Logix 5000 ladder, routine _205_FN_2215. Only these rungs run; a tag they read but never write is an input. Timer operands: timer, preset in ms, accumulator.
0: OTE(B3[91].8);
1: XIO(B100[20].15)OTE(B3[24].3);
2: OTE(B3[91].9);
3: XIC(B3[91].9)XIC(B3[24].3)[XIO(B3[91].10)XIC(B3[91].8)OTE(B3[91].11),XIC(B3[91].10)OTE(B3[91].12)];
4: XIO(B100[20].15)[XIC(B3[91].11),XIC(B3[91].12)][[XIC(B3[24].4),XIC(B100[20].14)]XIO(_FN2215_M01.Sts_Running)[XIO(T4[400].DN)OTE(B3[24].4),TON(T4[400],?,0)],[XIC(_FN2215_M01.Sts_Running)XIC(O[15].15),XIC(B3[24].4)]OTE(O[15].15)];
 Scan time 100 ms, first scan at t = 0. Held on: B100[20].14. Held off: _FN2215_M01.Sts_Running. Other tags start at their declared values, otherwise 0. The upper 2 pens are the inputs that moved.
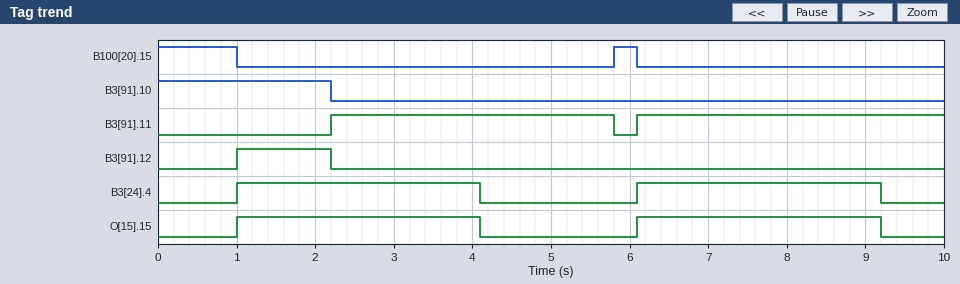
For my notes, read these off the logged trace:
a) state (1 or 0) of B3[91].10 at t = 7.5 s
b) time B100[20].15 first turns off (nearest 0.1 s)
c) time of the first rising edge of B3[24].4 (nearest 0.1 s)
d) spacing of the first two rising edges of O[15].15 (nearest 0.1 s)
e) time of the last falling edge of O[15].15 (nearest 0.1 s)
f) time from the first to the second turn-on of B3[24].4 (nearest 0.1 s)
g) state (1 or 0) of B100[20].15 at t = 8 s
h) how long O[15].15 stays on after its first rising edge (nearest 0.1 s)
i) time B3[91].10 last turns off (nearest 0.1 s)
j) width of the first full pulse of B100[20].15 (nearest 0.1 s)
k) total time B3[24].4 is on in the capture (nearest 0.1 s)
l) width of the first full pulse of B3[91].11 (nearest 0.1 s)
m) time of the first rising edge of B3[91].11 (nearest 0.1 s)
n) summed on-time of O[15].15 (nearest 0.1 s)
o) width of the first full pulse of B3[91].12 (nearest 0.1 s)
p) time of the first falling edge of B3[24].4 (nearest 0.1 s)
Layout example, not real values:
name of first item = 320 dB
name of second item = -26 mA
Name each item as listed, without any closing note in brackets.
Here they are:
state (1 or 0) of B3[91].10 at t = 7.5 s = 0
time B100[20].15 first turns off = 1.0 s
time of the first rising edge of B3[24].4 = 1.0 s
spacing of the first two rising edges of O[15].15 = 5.1 s
time of the last falling edge of O[15].15 = 9.2 s
time from the first to the second turn-on of B3[24].4 = 5.1 s
state (1 or 0) of B100[20].15 at t = 8 s = 0
how long O[15].15 stays on after its first rising edge = 3.1 s
time B3[91].10 last turns off = 2.2 s
width of the first full pulse of B100[20].15 = 0.3 s
total time B3[24].4 is on in the capture = 6.2 s
width of the first full pulse of B3[91].11 = 3.6 s
time of the first rising edge of B3[91].11 = 2.2 s
summed on-time of O[15].15 = 6.2 s
width of the first full pulse of B3[91].12 = 1.2 s
time of the first falling edge of B3[24].4 = 4.1 s
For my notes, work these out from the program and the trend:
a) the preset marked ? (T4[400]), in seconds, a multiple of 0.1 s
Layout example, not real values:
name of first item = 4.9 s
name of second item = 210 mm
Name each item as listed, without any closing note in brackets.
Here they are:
the preset marked ? (T4[400]), in seconds, a multiple of 0.1 s = 3.0 s
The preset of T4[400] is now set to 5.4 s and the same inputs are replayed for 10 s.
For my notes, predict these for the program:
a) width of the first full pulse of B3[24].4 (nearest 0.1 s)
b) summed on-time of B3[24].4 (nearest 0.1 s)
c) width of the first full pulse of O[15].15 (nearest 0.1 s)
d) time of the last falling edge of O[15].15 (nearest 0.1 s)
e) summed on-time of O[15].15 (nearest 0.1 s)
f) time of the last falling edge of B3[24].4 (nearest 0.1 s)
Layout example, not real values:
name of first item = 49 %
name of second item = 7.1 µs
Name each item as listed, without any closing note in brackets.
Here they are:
width of the first full pulse of B3[24].4 = 4.8 s
summed on-time of B3[24].4 = 8.7 s
width of the first full pulse of O[15].15 = 4.8 s
time of the last falling edge of O[15].15 = 5.8 s
summed on-time of O[15].15 = 8.7 s
time of the last falling edge of B3[24].4 = 5.8 s
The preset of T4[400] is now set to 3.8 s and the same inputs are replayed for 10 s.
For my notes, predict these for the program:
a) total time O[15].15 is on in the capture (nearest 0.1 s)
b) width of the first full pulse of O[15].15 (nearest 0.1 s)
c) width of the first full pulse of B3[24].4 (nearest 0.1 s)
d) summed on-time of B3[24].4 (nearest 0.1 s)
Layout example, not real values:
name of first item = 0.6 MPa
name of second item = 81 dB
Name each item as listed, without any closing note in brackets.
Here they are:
total time O[15].15 is on in the capture = 7.8 s
width of the first full pulse of O[15].15 = 3.9 s
width of the first full pulse of B3[24].4 = 3.9 s
summed on-time of B3[24].4 = 7.8 s
